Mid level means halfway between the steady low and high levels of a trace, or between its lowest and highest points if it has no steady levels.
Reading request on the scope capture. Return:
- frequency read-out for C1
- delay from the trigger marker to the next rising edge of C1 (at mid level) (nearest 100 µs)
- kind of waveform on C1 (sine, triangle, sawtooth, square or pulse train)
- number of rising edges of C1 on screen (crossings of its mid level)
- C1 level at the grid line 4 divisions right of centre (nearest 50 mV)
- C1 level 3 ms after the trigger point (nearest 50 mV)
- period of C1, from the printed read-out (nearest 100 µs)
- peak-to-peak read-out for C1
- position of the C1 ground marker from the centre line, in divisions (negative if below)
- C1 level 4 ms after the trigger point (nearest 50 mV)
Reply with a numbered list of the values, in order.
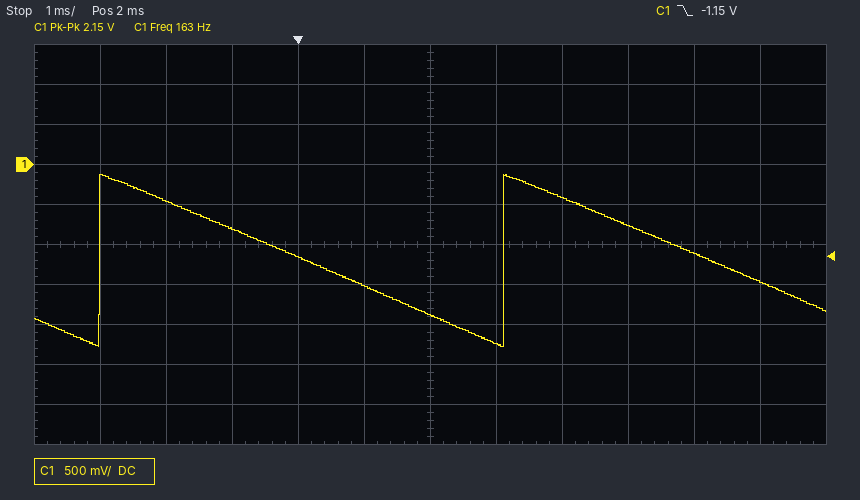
1. 163 Hz
2. 3.1 ms
3. sawtooth
4. 2
5. -1.10 V
6. -2.25 V
7. 6.1 ms
8. 2.15 V
9. +2.0 div
10. -400 mV
